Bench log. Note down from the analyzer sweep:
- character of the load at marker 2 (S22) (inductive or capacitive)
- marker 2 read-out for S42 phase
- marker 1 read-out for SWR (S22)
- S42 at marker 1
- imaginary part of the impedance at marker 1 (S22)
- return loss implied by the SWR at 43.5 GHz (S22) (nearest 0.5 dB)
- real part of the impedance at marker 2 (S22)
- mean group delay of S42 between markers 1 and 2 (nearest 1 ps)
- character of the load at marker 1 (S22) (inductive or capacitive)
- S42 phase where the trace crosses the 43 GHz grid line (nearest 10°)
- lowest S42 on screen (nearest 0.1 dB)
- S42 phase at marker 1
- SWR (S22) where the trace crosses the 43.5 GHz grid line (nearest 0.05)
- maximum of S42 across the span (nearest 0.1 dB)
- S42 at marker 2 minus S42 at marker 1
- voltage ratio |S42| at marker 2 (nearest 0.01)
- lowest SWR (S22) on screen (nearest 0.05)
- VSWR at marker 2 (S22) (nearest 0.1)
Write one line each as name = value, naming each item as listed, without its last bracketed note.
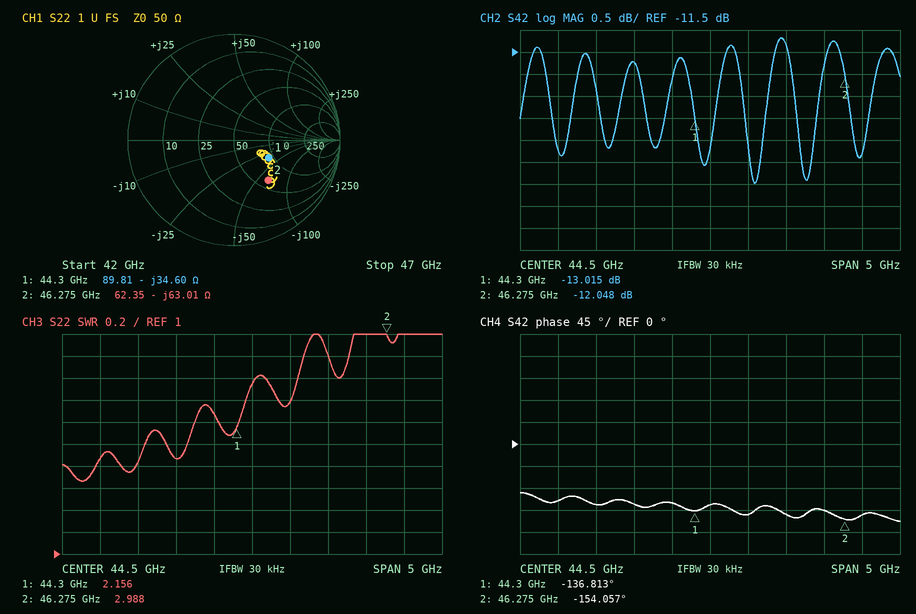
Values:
character of the load at marker 2 (S22) = capacitive
marker 2 read-out for S42 phase = -154.057°
marker 1 read-out for SWR = 2.156
S42 at marker 1 = -13.015 dB
imaginary part of the impedance at marker 1 = -34.60 Ω
return loss implied by the SWR at 43.5 GHz (S22) = 10.5 dB
real part of the impedance at marker 2 = 62.35 Ω
mean group delay of S42 between markers 1 and 2 = 24 ps
character of the load at marker 1 (S22) = capacitive
S42 phase where the trace crosses the 43 GHz grid line = -120°
lowest S42 on screen = -14.5 dB
S42 phase at marker 1 = -136.813°
SWR (S22) where the trace crosses the 43.5 GHz grid line = 1.85
maximum of S42 across the span = -11.2 dB
S42 at marker 2 minus S42 at marker 1 = 0.967 dB
voltage ratio |S42| at marker 2 = 0.25
lowest SWR (S22) on screen = 1.65
VSWR at marker 2 (S22) = 3.0
